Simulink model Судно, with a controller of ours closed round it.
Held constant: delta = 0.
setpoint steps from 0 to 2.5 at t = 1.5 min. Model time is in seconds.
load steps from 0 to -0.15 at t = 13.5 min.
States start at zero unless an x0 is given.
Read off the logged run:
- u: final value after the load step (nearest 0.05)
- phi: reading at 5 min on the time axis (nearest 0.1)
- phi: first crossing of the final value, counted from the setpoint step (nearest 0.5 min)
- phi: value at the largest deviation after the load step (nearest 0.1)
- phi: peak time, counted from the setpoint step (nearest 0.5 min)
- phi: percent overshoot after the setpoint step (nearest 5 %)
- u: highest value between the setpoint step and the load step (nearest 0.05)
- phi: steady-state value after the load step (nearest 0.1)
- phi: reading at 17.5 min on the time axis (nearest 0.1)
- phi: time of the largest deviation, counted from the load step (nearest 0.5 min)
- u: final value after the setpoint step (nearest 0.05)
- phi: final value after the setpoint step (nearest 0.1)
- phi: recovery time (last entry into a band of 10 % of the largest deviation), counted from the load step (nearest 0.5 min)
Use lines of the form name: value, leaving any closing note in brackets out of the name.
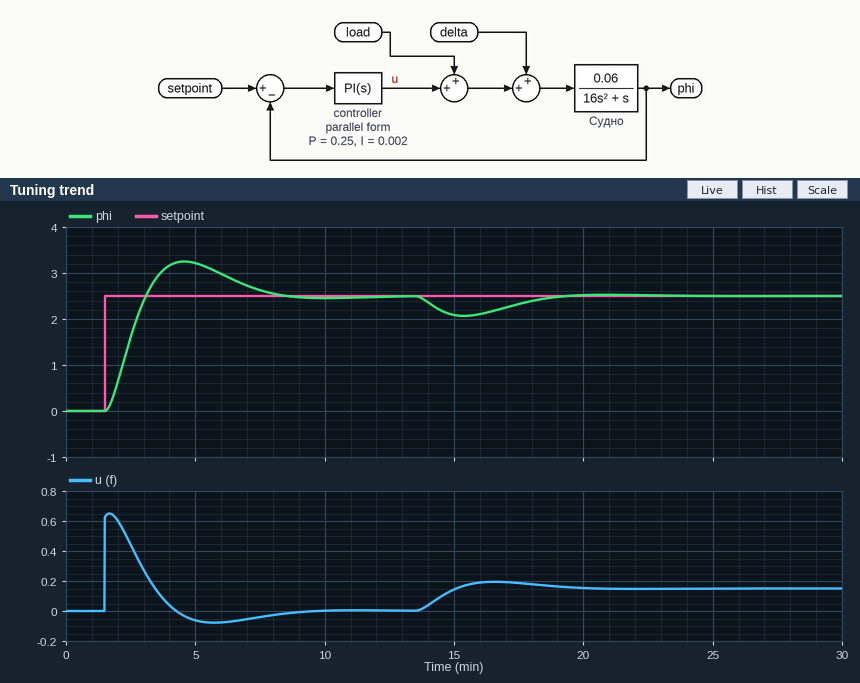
u: final value after the load step: 0.15
phi: reading at 5 min on the time axis: 3.2
phi: first crossing of the final value, counted from the setpoint step: 1.5 min
phi: value at the largest deviation after the load step: 2.1
phi: peak time, counted from the setpoint step: 3.0 min
phi: percent overshoot after the setpoint step: 30 %
u: highest value between the setpoint step and the load step: 0.65
phi: steady-state value after the load step: 2.5
phi: reading at 17.5 min on the time axis: 2.3
phi: time of the largest deviation, counted from the load step: 2.0 min
u: final value after the setpoint step: 0.00
phi: final value after the setpoint step: 2.5
phi: recovery time (last entry into a band of 10 % of the largest deviation), counted from the load step: 5.0 min
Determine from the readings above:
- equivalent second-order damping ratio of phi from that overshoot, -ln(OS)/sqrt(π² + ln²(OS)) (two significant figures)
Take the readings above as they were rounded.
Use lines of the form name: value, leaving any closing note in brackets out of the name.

equivalent second-order damping ratio of phi from that overshoot, -ln(OS)/sqrt(π² + ln²(OS)): 0.36
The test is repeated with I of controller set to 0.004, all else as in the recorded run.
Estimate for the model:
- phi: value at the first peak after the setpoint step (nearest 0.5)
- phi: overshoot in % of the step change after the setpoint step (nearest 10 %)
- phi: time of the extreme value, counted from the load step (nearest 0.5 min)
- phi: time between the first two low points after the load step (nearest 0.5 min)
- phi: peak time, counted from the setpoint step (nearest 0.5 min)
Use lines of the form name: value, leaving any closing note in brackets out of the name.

phi: value at the first peak after the setpoint step: 3.5
phi: overshoot in % of the step change after the setpoint step: 50 %
phi: time of the extreme value, counted from the load step: 1.5 min
phi: time between the first two low points after the load step: 6.5 min
phi: peak time, counted from the setpoint step: 2.5 min
